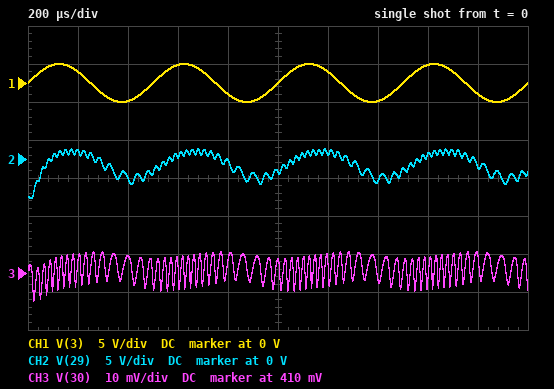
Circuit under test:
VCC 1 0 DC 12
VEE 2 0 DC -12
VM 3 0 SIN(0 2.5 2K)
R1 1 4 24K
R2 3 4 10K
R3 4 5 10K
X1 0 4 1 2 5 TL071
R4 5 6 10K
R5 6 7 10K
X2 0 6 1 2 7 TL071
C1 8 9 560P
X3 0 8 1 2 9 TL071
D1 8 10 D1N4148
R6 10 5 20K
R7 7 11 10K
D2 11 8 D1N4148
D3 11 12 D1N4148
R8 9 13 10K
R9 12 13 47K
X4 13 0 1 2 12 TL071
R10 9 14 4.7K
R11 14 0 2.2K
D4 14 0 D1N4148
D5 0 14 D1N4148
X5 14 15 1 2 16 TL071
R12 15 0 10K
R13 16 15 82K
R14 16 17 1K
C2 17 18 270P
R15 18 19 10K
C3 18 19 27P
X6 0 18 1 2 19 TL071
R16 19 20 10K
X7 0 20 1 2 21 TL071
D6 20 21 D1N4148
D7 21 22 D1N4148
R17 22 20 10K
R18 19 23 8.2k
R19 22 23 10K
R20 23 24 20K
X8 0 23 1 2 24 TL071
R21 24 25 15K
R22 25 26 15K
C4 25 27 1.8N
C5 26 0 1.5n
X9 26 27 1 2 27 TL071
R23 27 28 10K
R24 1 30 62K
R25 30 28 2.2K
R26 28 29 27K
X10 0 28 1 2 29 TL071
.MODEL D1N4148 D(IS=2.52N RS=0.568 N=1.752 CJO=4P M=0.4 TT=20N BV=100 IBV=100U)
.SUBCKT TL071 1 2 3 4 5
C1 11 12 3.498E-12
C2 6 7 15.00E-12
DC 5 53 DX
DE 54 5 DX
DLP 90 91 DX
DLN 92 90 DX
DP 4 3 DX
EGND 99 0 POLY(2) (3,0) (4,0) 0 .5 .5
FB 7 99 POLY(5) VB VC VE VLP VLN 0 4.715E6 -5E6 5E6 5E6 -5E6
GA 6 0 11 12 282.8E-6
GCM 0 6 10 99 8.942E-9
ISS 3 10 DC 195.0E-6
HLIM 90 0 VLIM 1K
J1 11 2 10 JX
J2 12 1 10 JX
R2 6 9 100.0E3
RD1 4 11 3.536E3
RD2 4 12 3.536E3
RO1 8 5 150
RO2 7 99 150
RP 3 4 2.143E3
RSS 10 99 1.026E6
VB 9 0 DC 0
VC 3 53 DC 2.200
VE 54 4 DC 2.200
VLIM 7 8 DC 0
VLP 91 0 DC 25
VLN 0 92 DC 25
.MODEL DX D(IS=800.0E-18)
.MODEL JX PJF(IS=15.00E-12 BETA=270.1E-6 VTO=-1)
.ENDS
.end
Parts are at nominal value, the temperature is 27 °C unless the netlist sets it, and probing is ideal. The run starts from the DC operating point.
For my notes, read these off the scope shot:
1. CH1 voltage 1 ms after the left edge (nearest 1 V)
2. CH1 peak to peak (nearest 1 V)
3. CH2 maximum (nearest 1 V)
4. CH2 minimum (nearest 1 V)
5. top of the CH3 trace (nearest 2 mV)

0 V
5 V
1 V
-5 V
416 mV
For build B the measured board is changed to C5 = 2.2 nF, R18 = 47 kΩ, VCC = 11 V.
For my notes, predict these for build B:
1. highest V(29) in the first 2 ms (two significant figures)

1.4 V
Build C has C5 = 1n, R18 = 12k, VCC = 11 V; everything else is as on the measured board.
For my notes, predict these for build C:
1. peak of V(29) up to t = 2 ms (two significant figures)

1.8 V
